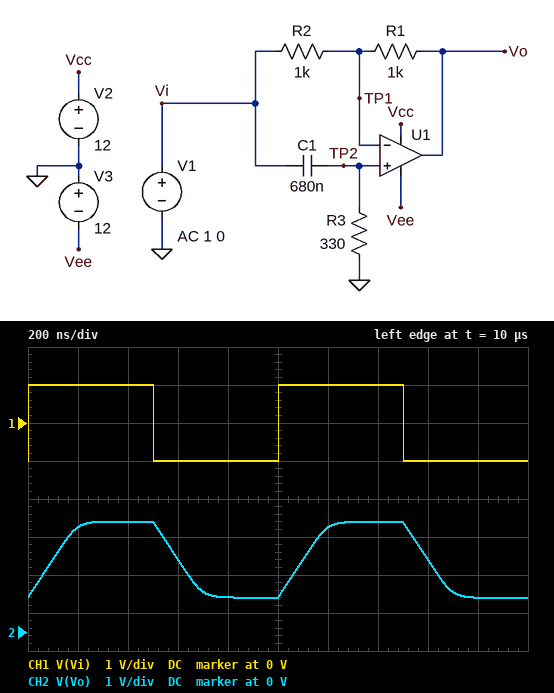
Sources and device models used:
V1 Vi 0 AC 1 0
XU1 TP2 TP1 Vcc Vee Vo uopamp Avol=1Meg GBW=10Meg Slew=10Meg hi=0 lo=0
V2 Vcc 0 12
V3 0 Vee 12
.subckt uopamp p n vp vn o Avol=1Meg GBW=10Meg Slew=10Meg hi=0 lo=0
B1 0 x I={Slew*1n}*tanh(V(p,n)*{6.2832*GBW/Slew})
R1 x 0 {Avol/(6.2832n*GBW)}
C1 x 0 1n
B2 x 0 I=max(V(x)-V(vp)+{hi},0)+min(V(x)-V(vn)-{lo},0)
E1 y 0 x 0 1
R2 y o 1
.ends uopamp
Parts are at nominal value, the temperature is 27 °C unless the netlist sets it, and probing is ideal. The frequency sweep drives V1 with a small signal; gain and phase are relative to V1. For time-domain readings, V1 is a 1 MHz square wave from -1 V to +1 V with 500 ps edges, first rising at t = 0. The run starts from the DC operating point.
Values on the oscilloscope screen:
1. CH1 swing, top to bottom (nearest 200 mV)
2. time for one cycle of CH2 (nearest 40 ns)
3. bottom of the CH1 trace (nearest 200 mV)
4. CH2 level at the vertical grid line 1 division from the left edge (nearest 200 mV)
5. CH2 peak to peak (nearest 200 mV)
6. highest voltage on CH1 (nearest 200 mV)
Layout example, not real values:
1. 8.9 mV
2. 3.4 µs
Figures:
1. 2.0 V
2. 1.00 µs
3. -1.0 V
4. 2.8 V
5. 2.0 V
6. 1.0 V
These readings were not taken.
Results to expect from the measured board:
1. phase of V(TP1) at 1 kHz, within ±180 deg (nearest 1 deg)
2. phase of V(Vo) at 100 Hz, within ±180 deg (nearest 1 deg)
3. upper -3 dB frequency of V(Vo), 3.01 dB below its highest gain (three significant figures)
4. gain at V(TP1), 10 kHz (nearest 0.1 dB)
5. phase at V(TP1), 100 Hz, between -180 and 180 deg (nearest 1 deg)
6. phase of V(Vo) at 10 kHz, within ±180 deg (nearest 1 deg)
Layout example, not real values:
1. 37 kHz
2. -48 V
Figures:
1. 35 deg
2. 164 deg
3. 5.00 MHz
4. 0 dB
5. 82 deg
6. 8 deg
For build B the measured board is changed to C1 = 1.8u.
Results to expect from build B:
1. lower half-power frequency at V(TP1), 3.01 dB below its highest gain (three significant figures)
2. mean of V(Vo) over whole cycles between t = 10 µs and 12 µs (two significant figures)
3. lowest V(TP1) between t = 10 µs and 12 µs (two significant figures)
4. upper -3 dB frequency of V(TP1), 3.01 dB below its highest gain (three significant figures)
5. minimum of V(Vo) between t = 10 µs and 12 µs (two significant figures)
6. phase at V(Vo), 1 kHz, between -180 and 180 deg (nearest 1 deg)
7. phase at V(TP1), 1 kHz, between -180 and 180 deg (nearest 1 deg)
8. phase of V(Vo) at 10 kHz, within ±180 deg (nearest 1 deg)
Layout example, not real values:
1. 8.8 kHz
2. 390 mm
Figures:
1. 268 Hz
2. 2.0 V
3. -20 mV
4. 7.07 MHz
5. 960 mV
6. 30 deg
7. 15 deg
8. 3 deg
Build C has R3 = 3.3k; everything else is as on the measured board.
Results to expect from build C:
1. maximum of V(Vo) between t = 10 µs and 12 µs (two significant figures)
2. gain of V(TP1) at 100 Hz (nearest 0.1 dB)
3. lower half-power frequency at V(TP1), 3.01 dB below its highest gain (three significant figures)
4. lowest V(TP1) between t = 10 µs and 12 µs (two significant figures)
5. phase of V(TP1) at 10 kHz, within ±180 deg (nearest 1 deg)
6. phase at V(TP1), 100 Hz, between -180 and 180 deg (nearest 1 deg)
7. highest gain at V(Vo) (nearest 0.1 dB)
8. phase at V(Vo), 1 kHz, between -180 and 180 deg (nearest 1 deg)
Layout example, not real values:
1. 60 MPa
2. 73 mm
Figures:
1. 3.0 V
2. -1.8 dB
3. 70.9 Hz
4. -5.3 mV
5. 0 deg
6. 35 deg
7. 0 dB
8. 8 deg
